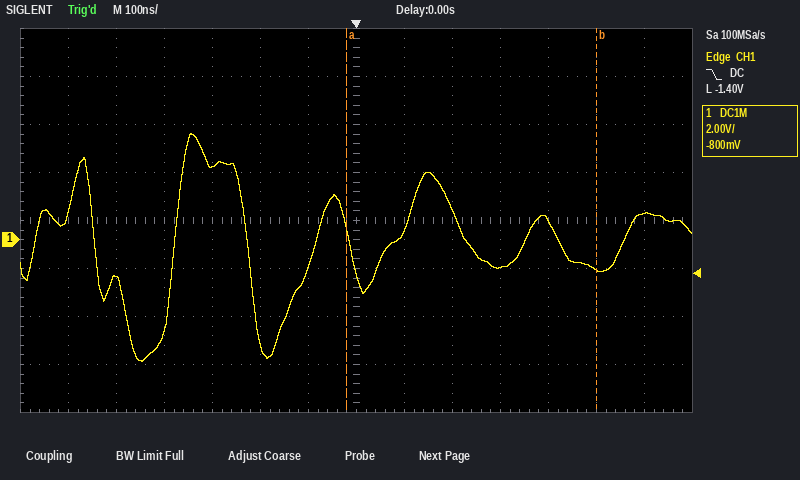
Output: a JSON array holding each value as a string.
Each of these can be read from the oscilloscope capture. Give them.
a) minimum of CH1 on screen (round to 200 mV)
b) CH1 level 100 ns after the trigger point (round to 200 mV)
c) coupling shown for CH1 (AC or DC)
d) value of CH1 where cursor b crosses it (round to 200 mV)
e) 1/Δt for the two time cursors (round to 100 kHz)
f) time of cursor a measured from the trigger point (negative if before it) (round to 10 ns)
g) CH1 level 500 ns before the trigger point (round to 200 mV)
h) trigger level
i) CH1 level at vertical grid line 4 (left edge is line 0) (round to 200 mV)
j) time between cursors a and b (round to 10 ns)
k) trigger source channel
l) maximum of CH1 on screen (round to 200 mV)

["-5.0 V", "400 mV", "DC", "-1.2 V", "1.9 MHz", "-20 ns", "-1.6 V", "-1.40 V", "3.0 V", "520 ns", "CH1", "4.4 V"]
